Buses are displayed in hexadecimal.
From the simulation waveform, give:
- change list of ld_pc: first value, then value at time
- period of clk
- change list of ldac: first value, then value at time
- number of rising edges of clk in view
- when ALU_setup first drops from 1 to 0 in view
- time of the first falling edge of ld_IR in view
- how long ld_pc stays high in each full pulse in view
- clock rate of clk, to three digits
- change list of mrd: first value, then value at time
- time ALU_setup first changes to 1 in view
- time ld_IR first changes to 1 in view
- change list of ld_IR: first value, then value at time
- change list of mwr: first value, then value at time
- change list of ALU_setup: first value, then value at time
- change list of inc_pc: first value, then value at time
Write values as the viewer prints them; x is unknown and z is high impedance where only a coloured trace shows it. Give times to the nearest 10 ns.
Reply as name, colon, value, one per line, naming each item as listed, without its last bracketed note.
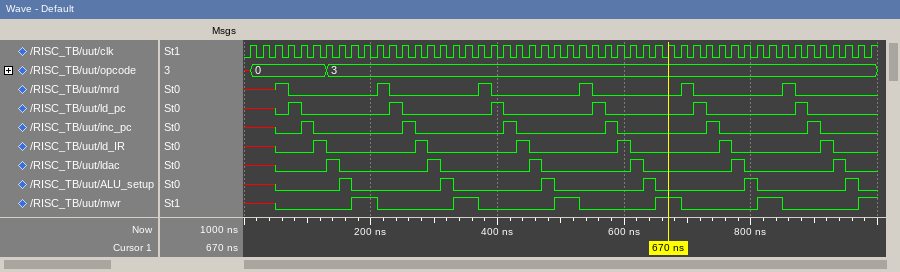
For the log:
change list of ld_pc: first value, then value at time: x, 0 at 50 ns, 1 at 70 ns, 0 at 90 ns, 1 at 230 ns, 0 at 250 ns, 1 at 390 ns, 0 at 410 ns, 1 at 550 ns, 0 at 570 ns, 1 at 710 ns, 0 at 730 ns, 1 at 870 ns, 0 at 890 ns
period of clk: 20 ns
change list of ldac: first value, then value at time: x, 0 at 50 ns, 1 at 130 ns, 0 at 150 ns, 1 at 290 ns, 0 at 310 ns, 1 at 450 ns, 0 at 470 ns, 1 at 610 ns, 0 at 630 ns, 1 at 770 ns, 0 at 790 ns, 1 at 930 ns, 0 at 950 ns
number of rising edges of clk in view: 50
when ALU_setup first drops from 1 to 0 in view: 170 ns
time of the first falling edge of ld_IR in view: 130 ns
how long ld_pc stays high in each full pulse in view: 20 ns, 20 ns, 20 ns, 20 ns, 20 ns, 20 ns
clock rate of clk, to three digits: 50.0 MHz
change list of mrd: first value, then value at time: x, 1 at 50 ns, 0 at 70 ns, 1 at 210 ns, 0 at 230 ns, 1 at 370 ns, 0 at 390 ns, 1 at 530 ns, 0 at 550 ns, 1 at 690 ns, 0 at 710 ns, 1 at 850 ns, 0 at 870 ns
time ALU_setup first changes to 1 in view: 150 ns
time ld_IR first changes to 1 in view: 110 ns
change list of ld_IR: first value, then value at time: x, 0 at 50 ns, 1 at 110 ns, 0 at 130 ns, 1 at 270 ns, 0 at 290 ns, 1 at 430 ns, 0 at 450 ns, 1 at 590 ns, 0 at 610 ns, 1 at 750 ns, 0 at 770 ns, 1 at 910 ns, 0 at 930 ns
change list of mwr: first value, then value at time: x, 0 at 50 ns, 1 at 170 ns, 0 at 210 ns, 1 at 330 ns, 0 at 370 ns, 1 at 490 ns, 0 at 530 ns, 1 at 650 ns, 0 at 690 ns, 1 at 810 ns, 0 at 850 ns, 1 at 970 ns
change list of ALU_setup: first value, then value at time: x, 0 at 50 ns, 1 at 150 ns, 0 at 170 ns, 1 at 310 ns, 0 at 330 ns, 1 at 470 ns, 0 at 490 ns, 1 at 630 ns, 0 at 650 ns, 1 at 790 ns, 0 at 810 ns, 1 at 950 ns, 0 at 970 ns
change list of inc_pc: first value, then value at time: x, 0 at 50 ns, 1 at 90 ns, 0 at 110 ns, 1 at 250 ns, 0 at 270 ns, 1 at 410 ns, 0 at 430 ns, 1 at 570 ns, 0 at 590 ns, 1 at 730 ns, 0 at 750 ns, 1 at 890 ns, 0 at 910 ns
